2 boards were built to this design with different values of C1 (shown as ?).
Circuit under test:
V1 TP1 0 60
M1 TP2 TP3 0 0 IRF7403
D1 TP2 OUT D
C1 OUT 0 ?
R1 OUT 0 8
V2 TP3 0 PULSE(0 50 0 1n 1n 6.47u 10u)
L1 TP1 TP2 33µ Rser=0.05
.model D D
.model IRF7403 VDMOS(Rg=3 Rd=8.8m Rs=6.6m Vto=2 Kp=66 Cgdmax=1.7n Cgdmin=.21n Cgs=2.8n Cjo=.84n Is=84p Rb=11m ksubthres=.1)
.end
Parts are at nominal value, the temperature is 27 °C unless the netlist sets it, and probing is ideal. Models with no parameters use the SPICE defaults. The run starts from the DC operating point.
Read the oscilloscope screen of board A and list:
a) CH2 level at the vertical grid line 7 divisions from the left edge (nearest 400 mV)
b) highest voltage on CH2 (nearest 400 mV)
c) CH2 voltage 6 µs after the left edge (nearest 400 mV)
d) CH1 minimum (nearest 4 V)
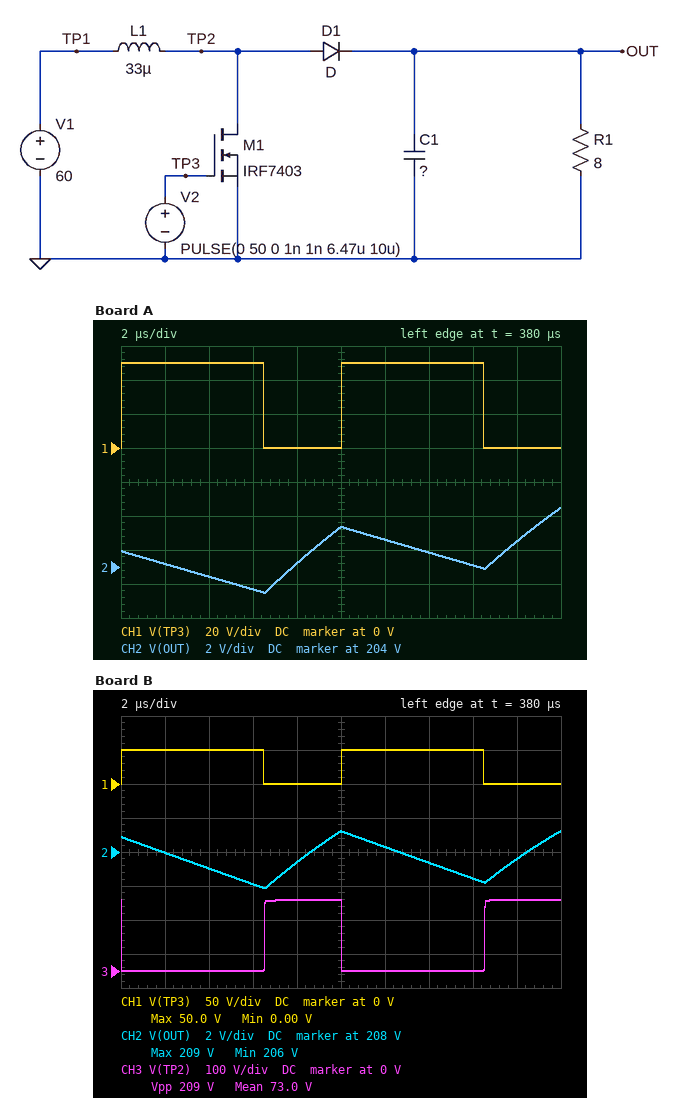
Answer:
204.8 V
207.6 V
202.8 V
0 V
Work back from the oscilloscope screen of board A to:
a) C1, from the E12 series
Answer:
68 µF
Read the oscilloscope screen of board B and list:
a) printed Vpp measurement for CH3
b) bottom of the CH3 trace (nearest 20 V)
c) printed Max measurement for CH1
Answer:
209 V
0 V
50.0 V
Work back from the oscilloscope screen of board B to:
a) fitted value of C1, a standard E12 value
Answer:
56 µF
